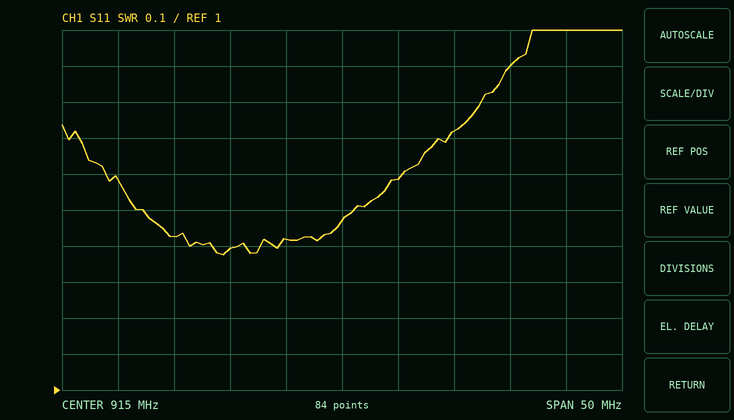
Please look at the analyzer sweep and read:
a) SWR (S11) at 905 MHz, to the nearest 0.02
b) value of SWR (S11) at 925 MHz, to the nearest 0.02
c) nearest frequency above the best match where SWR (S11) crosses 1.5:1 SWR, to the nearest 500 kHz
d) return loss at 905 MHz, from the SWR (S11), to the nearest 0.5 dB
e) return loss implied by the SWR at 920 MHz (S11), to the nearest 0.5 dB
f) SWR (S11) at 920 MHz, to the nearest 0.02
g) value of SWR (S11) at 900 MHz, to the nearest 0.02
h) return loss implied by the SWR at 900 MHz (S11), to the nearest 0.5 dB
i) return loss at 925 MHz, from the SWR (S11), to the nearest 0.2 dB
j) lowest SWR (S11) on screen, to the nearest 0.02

1.40
1.72
916.0 MHz
15.5 dB
13.0 dB
1.58
1.42
15.0 dB
11.6 dB
1.38
